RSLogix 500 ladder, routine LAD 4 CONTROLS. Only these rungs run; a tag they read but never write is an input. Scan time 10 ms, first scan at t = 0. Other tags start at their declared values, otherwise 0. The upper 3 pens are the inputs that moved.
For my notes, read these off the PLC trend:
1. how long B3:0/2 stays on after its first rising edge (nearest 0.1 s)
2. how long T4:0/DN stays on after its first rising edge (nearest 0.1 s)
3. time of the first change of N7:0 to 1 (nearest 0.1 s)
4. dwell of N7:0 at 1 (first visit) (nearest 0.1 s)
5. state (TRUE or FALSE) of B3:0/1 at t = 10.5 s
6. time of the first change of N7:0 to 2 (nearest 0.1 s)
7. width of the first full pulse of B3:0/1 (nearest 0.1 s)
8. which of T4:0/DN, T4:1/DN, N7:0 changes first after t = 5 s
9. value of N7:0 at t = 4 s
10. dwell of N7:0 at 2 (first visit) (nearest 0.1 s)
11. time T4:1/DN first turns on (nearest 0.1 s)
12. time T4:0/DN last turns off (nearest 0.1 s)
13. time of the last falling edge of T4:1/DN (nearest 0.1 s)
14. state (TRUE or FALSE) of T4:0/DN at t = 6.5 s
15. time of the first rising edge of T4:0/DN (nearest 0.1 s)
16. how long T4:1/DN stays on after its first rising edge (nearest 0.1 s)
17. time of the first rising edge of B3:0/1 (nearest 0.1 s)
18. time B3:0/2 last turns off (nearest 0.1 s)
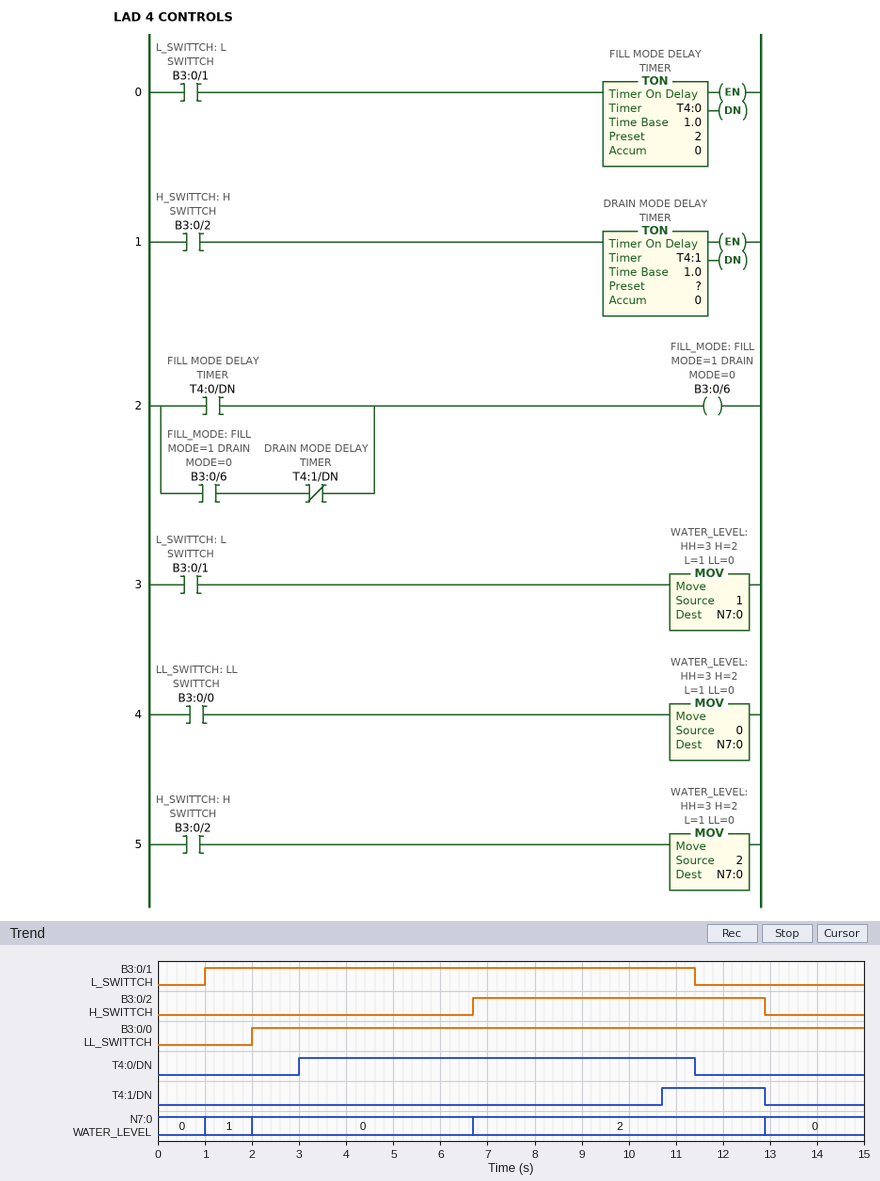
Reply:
6.2 s
8.4 s
1.0 s
1.0 s
TRUE
6.7 s
10.4 s
N7:0
0
6.2 s
10.7 s
11.4 s
12.9 s
TRUE
3.0 s
2.2 s
1.0 s
12.9 s
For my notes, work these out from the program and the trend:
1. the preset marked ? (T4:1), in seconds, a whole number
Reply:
4 s
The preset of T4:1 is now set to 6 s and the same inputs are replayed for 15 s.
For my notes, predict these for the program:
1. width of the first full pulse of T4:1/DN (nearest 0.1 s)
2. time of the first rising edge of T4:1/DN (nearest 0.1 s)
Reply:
0.2 s
12.7 s
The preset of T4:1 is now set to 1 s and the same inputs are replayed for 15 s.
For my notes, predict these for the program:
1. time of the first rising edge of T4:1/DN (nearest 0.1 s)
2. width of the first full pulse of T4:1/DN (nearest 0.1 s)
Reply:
7.7 s
5.2 s
